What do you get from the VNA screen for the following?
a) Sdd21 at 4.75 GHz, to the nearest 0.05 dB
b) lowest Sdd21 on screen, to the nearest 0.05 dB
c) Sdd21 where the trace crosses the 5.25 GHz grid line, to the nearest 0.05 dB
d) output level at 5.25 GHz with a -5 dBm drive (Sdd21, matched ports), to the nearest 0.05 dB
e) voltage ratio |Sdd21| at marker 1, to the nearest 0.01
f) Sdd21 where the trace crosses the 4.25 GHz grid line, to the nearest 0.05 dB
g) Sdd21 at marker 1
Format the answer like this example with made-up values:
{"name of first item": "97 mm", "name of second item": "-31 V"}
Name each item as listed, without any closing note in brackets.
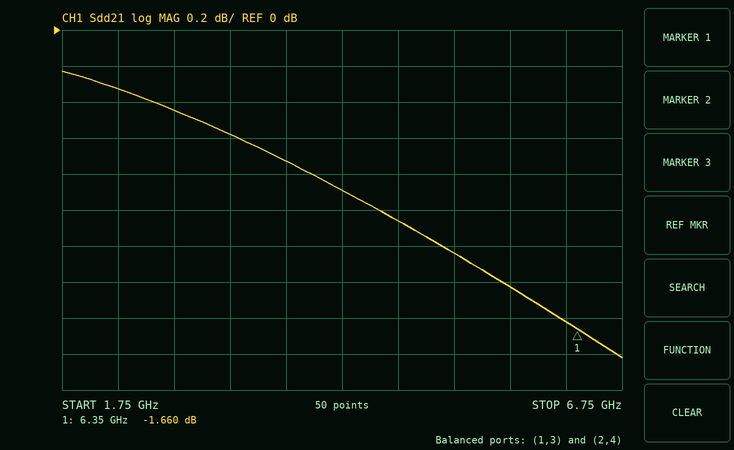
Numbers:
{"Sdd21 at 4.75 GHz, to the nearest 0.05 dB": "-1.05 dB", "lowest Sdd21 on screen, to the nearest 0.05 dB": "-1.80 dB", "Sdd21 where the trace crosses the 5.25 GHz grid line, to the nearest 0.05 dB": "-1.25 dB", "output level at 5.25 GHz with a -5 dBm drive (Sdd21, matched ports), to the nearest 0.05 dB": "-6.25 dBm", "voltage ratio |Sdd21| at marker 1, to the nearest 0.01": "0.83", "Sdd21 where the trace crosses the 4.25 GHz grid line, to the nearest 0.05 dB": "-0.90 dB", "Sdd21 at marker 1": "-1.660 dB"}
